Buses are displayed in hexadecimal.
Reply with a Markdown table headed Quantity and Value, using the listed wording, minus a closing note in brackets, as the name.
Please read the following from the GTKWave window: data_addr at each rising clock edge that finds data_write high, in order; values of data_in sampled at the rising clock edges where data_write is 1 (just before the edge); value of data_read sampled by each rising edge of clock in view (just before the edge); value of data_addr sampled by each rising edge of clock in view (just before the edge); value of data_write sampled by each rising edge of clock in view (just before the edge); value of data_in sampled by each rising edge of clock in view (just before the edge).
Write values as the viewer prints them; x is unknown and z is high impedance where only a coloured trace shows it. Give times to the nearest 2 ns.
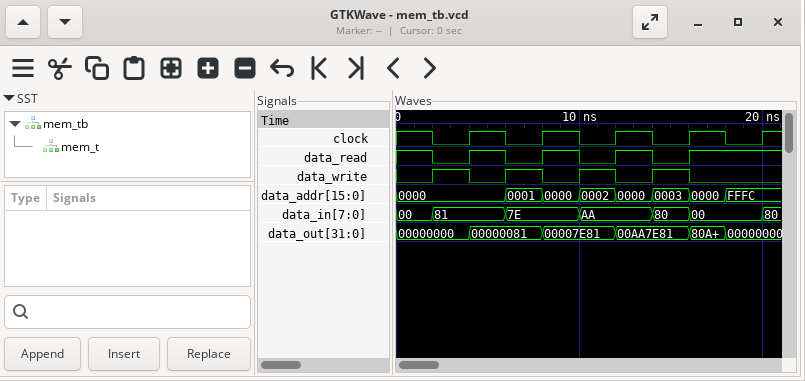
| Quantity | Value |
|---|---|
| data_addr at each rising clock edge that finds data_write high, in order | 0000, 0001, 0002, 0003 |
| values of data_in sampled at the rising clock edges where data_write is 1 | 81, 7E, AA, 80 |
| value of data_read sampled by each rising edge of clock in view | 0 0 0 0 1 |
| value of data_addr sampled by each rising edge of clock in view | 0000, 0001, 0002, 0003, FFFC |
| value of data_write sampled by each rising edge of clock in view | 1 1 1 1 0 |
| value of data_in sampled by each rising edge of clock in view | 81, 7E, AA, 80, 00 |
